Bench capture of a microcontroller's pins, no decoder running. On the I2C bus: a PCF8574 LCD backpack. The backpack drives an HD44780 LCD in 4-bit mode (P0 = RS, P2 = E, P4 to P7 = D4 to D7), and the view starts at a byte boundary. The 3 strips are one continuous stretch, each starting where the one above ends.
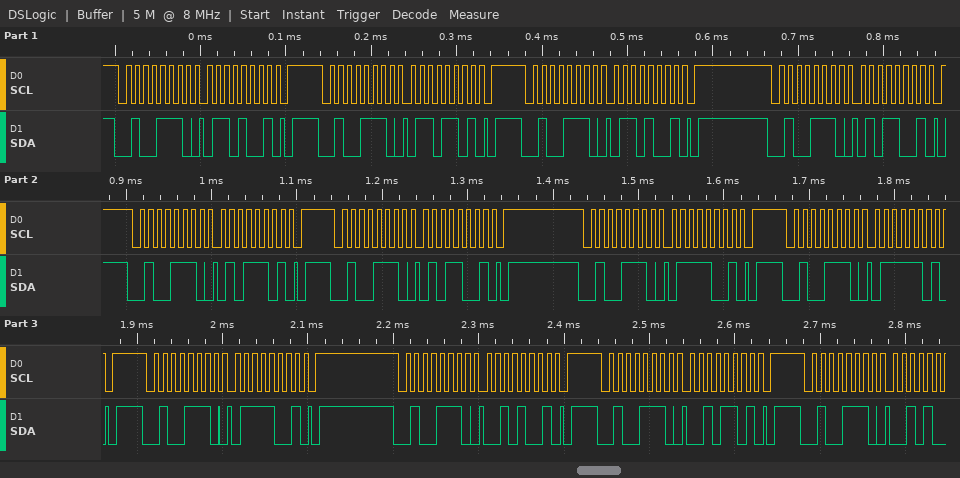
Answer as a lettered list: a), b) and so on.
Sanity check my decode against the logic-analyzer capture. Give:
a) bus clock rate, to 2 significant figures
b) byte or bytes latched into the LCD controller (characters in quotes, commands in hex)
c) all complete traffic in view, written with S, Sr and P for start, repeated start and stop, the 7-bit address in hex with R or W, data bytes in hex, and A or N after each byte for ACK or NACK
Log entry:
a) 100 kHz
b) 'e'
c) S 27W A 69 A P S 27W A 6D A P S 27W A 69 A P S 27W A 59 A P S 27W A 5D A P S 27W A 59 A P S 27W A 79 A P S 27W A 7D A P S 27W A 79 A P S 27W A 29 A P S 27W A 2D A P S 27W A
